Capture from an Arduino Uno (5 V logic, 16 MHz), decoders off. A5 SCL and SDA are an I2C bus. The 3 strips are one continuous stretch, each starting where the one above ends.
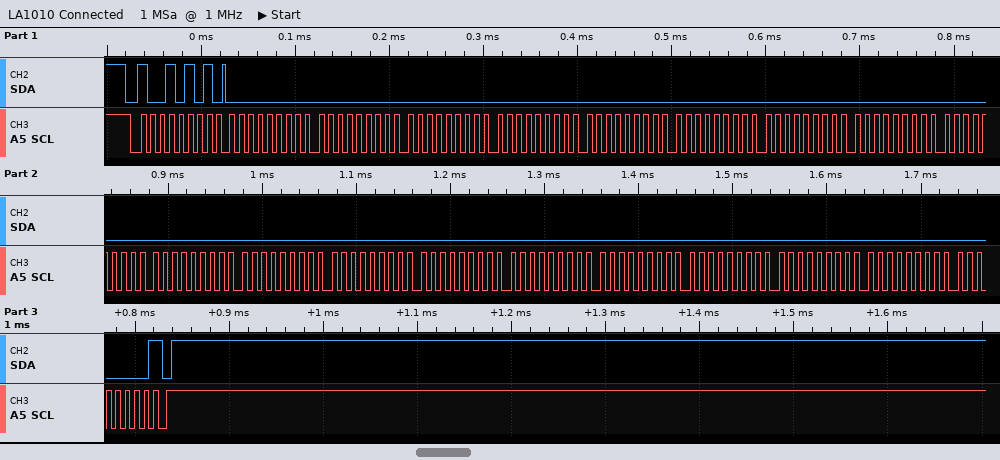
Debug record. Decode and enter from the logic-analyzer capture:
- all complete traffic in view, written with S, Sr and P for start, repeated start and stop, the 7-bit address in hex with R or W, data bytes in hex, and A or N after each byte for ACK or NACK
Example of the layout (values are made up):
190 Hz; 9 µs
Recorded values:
S 4AR A 00 A 00 A 00 A 00 A 00 A 00 A 00 A 00 A 00 A 00 A 00 A 00 A 00 A 00 A 00 A 00 A 00 A 00 A 00 N P
